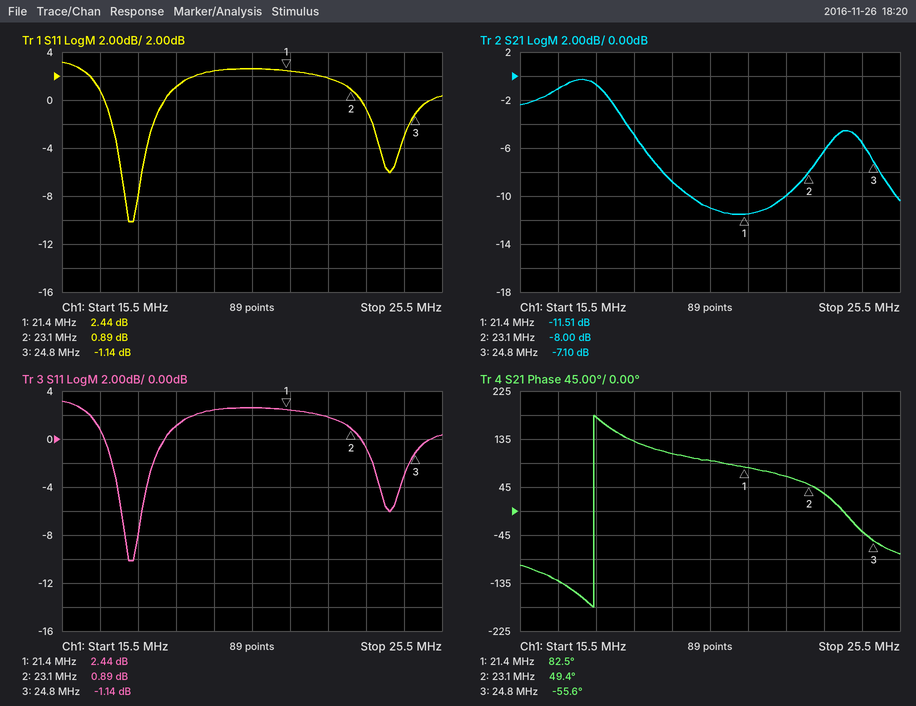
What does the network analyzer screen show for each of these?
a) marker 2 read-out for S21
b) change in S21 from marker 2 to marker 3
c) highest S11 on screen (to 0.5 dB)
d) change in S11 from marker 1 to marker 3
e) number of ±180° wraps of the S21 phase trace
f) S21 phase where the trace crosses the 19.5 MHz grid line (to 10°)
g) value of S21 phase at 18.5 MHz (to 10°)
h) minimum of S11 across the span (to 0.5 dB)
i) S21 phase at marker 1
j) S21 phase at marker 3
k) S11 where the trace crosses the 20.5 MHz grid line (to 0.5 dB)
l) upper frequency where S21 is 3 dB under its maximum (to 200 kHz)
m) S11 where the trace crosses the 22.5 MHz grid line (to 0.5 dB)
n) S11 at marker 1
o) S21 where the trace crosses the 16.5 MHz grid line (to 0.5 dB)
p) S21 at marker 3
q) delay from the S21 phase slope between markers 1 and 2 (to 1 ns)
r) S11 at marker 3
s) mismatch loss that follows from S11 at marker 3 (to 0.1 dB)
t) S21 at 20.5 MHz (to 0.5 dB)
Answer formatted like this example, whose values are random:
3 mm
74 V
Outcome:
-8.00 dB
0.90 dB
3.0 dB
-3.58 dB
1
110°
130°
-10.0 dB
82.5°
-55.6°
2.5 dB
18.2 MHz
2.0 dB
2.44 dB
-1.0 dB
-7.10 dB
54 ns
-1.14 dB
6.4 dB
-11.0 dB
